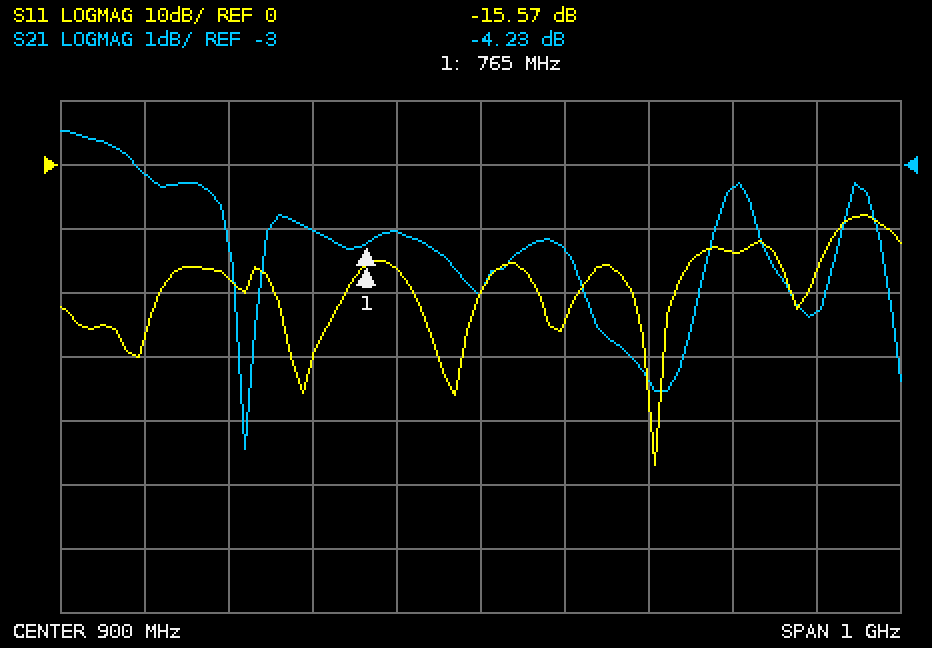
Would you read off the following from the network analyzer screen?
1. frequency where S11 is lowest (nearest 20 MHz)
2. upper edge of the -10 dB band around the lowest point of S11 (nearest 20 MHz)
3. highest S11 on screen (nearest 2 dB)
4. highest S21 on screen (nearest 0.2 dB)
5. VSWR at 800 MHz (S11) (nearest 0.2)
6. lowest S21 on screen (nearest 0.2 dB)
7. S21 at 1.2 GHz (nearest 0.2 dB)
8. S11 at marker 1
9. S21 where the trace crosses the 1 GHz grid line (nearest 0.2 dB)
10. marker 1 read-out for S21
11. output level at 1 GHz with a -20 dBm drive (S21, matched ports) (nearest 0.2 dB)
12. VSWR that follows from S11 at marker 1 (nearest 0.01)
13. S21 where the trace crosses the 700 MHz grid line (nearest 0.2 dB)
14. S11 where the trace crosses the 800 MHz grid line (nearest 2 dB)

1.10 GHz
1.32 GHz
-8 dB
-2.4 dB
1.4
-7.4 dB
-3.4 dB
-15.57 dB
-4.4 dB
-4.23 dB
-24.4 dBm
1.40
-4.0 dB
-16 dB
